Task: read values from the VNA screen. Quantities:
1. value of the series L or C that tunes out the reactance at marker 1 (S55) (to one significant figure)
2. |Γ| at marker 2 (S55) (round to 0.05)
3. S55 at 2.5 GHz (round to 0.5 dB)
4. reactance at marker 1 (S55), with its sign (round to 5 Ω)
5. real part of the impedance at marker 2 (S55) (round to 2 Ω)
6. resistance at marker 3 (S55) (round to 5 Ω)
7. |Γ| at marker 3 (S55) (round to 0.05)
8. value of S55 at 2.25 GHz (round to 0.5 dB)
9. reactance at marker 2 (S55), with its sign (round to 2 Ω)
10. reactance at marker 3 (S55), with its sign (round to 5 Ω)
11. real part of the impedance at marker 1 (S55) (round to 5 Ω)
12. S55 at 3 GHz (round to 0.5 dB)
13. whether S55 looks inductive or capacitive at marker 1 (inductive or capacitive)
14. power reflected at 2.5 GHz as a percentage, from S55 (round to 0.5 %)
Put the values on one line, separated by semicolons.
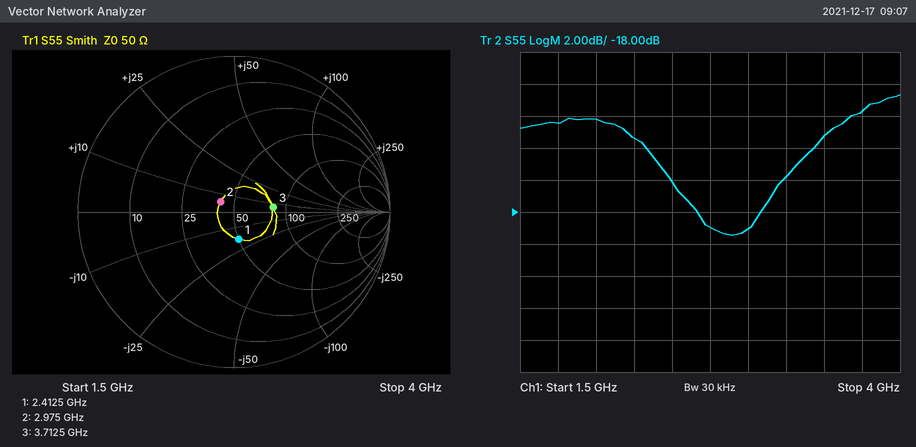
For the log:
1 nH; 0.10; -16.0 dB; -20 Ω; 42 Ω; 85 Ω; 0.25; -13.5 dB; +6 Ω; +5 Ω; 50 Ω; -19.0 dB; capacitive; 2.5 %
